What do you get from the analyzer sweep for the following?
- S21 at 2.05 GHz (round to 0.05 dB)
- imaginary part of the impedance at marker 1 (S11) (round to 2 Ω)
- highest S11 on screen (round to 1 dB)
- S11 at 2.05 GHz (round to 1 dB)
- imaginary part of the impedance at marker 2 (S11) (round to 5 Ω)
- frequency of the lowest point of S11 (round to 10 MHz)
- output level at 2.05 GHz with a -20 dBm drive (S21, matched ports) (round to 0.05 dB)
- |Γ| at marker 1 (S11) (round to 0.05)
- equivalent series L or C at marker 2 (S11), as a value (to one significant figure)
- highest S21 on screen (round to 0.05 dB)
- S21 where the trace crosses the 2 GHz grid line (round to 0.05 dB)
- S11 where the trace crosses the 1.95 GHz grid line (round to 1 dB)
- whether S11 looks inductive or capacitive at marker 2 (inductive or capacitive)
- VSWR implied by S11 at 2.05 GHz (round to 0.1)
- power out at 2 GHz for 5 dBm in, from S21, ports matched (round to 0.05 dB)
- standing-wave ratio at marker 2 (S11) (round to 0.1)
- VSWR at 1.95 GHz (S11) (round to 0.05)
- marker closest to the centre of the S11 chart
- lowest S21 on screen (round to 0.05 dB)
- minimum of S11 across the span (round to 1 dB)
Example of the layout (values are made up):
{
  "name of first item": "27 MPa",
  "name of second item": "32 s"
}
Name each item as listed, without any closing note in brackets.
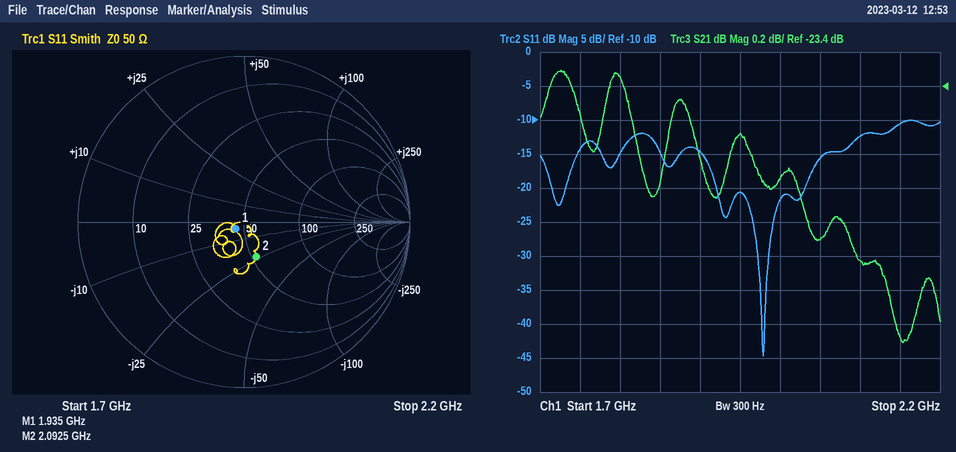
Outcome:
{
  "S21 at 2.05 GHz": "-24.30 dB",
  "imaginary part of the impedance at marker 1 (S11)": "-4 Ω",
  "highest S11 on screen": "-10 dB",
  "S11 at 2.05 GHz": "-16 dB",
  "imaginary part of the impedance at marker 2 (S11)": "-25 Ω",
  "frequency of the lowest point of S11": "1.98 GHz",
  "output level at 2.05 GHz with a -20 dBm drive (S21, matched ports)": "-44.30 dBm",
  "|Γ| at marker 1 (S11)": "0.05",
  "equivalent series L or C at marker 2 (S11), as a value": "3 pF",
  "highest S21 on screen": "-23.30 dB",
  "S21 where the trace crosses the 2 GHz grid line": "-23.95 dB",
  "S11 where the trace crosses the 1.95 GHz grid line": "-21 dB",
  "whether S11 looks inductive or capacitive at marker 2": "capacitive",
  "VSWR implied by S11 at 2.05 GHz": "1.4",
  "power out at 2 GHz for 5 dBm in, from S21, ports matched": "-18.95 dBm",
  "standing-wave ratio at marker 2 (S11)": "1.6",
  "VSWR at 1.95 GHz (S11)": "1.20",
  "marker closest to the centre of the S11 chart": "marker 1",
  "lowest S21 on screen": "-24.90 dB",
  "minimum of S11 across the span": "-45 dB"
}
